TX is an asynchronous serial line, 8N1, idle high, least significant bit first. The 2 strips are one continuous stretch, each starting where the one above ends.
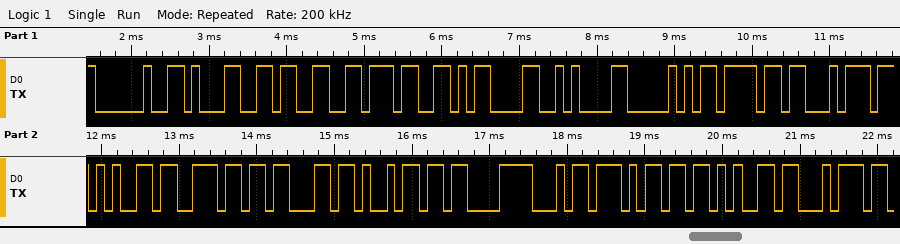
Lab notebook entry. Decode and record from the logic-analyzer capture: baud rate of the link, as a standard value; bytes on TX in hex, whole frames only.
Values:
9600 baud
20 31 33 37 0D 0A 50 6F 74 65 6E 63 69 C3 B4 6D 65 74
